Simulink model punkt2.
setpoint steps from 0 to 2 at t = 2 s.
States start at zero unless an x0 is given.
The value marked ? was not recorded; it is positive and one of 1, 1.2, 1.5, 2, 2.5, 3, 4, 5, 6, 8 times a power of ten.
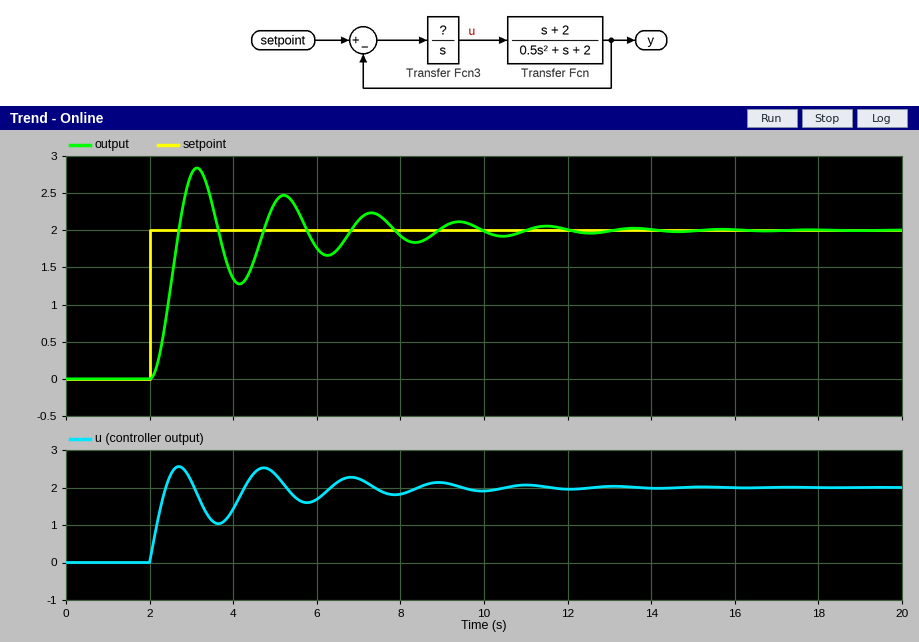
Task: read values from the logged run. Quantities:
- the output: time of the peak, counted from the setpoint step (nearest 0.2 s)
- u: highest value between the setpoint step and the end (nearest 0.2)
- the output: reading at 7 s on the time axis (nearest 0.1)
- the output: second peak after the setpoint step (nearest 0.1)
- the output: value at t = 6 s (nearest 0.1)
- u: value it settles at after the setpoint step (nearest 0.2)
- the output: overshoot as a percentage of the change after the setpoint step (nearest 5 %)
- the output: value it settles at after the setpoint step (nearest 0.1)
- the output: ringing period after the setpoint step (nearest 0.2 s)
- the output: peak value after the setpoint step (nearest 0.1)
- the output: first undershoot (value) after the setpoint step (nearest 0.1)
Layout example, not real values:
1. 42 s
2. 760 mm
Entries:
1. 1.2 s
2. 2.6
3. 2.1
4. 2.5
5. 1.8
6. 2.0
7. 40 %
8. 2.0
9. 2.0 s
10. 2.8
11. 1.3
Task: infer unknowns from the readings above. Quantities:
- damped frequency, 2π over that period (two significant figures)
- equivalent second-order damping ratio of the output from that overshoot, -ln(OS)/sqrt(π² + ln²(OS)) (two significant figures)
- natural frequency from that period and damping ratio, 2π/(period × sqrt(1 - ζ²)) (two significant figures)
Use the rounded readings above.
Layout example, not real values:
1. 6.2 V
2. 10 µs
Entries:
1. 3.1 rad/s
2. 0.28
3. 3.3 rad/s
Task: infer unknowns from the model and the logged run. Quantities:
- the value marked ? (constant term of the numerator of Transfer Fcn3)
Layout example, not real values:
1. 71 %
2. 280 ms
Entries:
1. 3
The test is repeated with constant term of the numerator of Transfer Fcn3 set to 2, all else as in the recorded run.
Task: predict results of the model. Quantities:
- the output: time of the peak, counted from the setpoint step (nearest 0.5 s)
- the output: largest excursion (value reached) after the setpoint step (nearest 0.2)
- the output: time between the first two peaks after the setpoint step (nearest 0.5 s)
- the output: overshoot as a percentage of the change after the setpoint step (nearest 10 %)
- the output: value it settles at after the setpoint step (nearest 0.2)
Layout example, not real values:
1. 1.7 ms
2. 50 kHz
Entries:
1. 1.5 s
2. 2.6
3. 2.5 s
4. 30 %
5. 2.0
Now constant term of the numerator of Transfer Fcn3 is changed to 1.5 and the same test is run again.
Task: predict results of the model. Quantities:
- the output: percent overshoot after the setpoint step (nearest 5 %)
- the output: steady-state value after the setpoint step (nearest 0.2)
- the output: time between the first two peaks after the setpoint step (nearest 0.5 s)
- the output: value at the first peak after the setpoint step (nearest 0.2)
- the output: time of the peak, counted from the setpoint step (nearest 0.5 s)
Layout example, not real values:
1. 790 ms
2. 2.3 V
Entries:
1. 15 %
2. 2.0
3. 2.5 s
4. 2.4
5. 1.5 s
